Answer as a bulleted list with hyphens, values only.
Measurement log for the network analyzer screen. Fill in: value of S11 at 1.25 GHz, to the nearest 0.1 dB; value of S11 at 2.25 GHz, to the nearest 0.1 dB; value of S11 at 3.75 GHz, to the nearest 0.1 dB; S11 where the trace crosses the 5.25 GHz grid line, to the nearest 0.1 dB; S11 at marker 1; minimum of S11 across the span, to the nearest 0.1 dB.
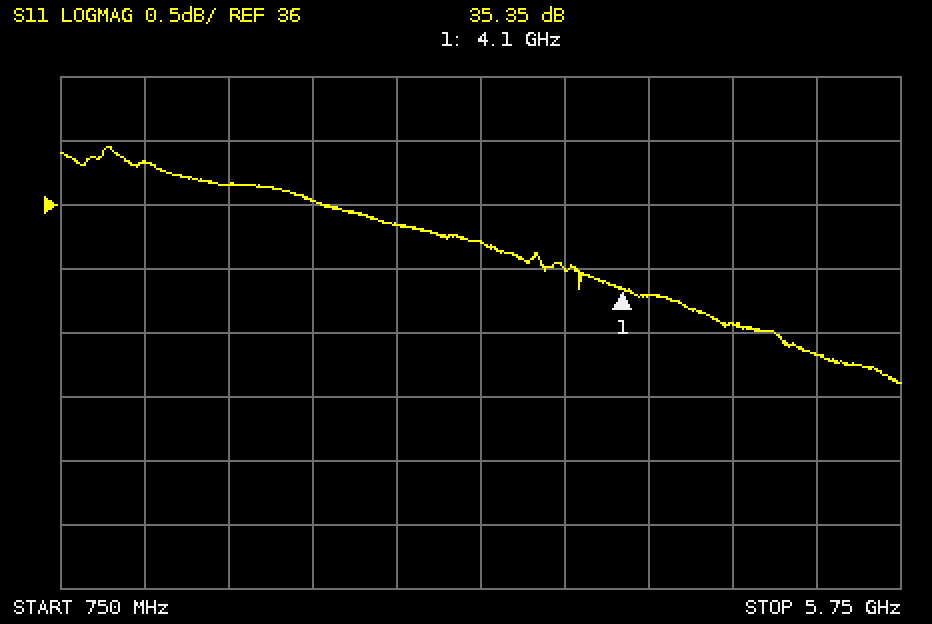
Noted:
- 36.3 dB
- 36.0 dB
- 35.5 dB
- 34.8 dB
- 35.35 dB
- 34.6 dB
